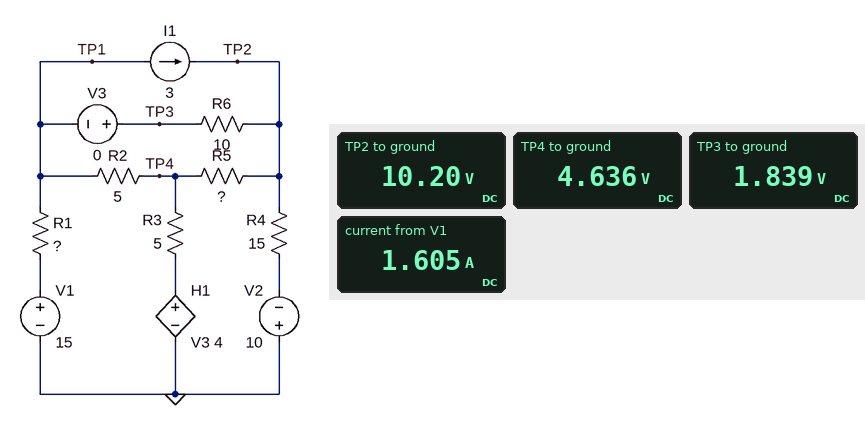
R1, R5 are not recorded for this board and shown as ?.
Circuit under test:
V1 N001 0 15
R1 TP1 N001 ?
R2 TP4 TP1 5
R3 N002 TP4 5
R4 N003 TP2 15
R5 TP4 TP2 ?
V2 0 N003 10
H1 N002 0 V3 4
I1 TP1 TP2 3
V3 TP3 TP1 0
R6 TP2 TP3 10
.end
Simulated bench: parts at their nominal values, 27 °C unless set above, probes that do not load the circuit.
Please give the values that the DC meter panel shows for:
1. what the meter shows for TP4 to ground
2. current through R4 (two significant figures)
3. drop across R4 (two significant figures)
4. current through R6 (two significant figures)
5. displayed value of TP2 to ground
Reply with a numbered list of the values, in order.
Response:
1. 4.636 V
2. 1.3 A
3. 20 V
4. 840 mA
5. 10.20 V
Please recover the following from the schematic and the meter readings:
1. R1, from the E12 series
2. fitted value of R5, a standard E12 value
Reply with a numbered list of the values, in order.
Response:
1. 8.2 Ω
2. 6.8 Ω
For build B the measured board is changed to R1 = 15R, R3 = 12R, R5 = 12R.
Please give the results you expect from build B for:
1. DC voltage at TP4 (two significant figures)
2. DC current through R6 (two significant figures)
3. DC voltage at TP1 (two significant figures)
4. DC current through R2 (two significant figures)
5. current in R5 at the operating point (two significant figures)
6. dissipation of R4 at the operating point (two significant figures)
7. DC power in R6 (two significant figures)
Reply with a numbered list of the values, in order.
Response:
1. 2.2 V
2. 1.1 A
3. -1.7 V
4. 780 mA
5. 600 mA
6. 25 W
7. 12 W
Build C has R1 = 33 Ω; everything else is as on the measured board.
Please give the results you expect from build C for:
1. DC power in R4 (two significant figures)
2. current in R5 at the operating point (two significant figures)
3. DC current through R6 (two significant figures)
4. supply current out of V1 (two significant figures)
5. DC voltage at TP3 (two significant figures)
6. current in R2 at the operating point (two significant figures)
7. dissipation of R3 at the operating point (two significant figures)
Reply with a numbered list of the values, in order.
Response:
1. 19 W
2. 740 mA
3. 1.1 A
4. 590 mA
5. -4.5 V
6. 1.3 A
7. 1.4 W
